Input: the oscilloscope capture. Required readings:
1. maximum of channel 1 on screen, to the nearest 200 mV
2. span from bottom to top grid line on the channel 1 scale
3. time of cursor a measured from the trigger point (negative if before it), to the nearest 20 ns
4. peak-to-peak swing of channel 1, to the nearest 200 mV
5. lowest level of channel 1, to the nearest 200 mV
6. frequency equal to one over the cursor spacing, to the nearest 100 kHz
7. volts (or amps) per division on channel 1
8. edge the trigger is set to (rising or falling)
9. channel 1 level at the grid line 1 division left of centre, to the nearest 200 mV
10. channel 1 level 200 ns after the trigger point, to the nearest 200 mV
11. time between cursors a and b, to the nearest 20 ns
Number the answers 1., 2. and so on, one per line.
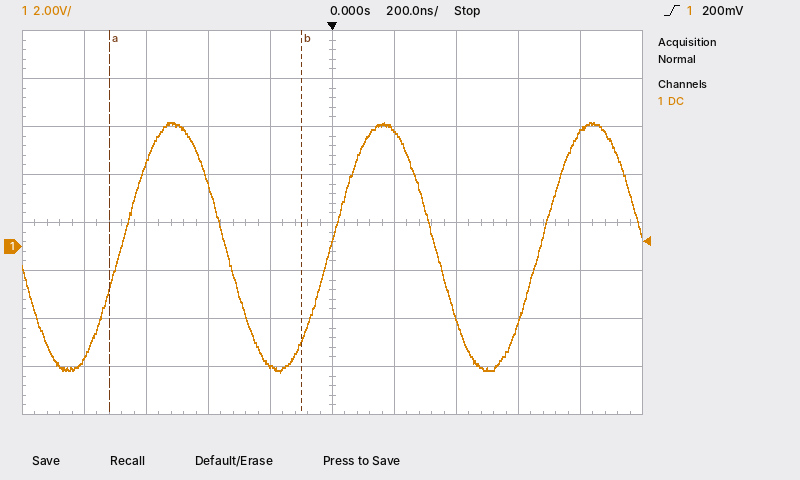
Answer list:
1. 5.2 V
2. 16 V
3. -720 ns
4. 10.4 V
5. -5.2 V
6. 1.6 MHz
7. 2 V
8. rising
9. -5.0 V
10. 4.8 V
11. 620 ns
